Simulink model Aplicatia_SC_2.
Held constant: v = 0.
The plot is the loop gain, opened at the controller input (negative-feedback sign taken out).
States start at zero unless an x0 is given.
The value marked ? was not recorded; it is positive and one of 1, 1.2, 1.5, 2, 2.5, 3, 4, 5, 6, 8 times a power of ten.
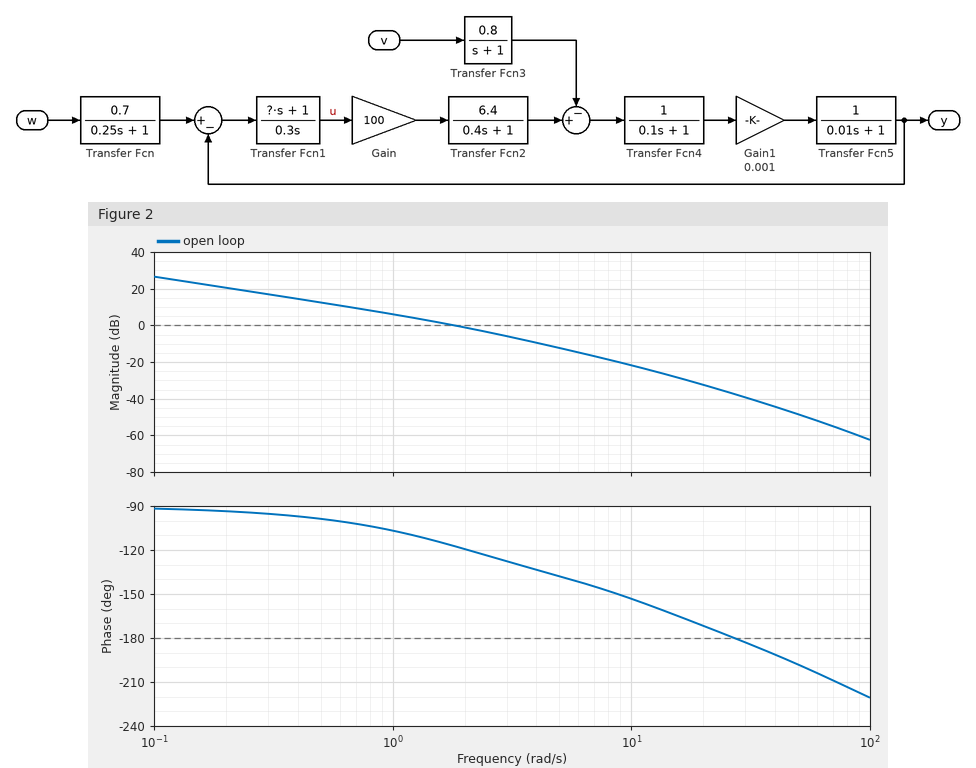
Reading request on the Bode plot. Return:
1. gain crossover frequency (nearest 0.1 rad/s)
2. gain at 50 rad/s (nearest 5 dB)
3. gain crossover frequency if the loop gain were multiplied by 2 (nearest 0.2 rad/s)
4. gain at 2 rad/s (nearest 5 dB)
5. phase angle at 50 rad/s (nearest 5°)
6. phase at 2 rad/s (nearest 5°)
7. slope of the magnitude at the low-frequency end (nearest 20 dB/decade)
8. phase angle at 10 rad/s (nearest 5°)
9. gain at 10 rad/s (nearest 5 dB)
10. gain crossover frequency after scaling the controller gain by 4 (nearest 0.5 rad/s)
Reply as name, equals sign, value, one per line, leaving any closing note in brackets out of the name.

gain crossover frequency = 1.8 rad/s
gain at 50 rad/s = -50 dB
gain crossover frequency if the loop gain were multiplied by 2 = 3.0 rad/s
gain at 2 rad/s = 0 dB
phase angle at 50 rad/s = -200°
phase at 2 rad/s = -120°
slope of the magnitude at the low-frequency end = -20 dB/decade
phase angle at 10 rad/s = -155°
gain at 10 rad/s = -20 dB
gain crossover frequency after scaling the controller gain by 4 = 5.0 rad/s
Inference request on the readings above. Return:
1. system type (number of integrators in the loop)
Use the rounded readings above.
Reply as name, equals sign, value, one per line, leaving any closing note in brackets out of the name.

system type = 1
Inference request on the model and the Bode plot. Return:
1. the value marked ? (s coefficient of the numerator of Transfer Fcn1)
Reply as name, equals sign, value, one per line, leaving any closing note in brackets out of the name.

the value marked ? = 0.2
